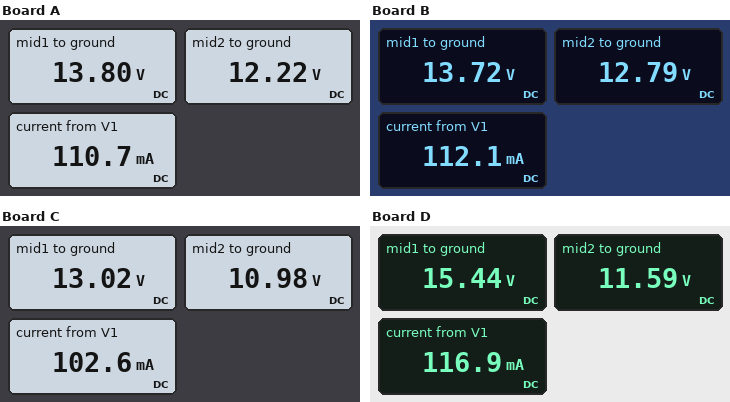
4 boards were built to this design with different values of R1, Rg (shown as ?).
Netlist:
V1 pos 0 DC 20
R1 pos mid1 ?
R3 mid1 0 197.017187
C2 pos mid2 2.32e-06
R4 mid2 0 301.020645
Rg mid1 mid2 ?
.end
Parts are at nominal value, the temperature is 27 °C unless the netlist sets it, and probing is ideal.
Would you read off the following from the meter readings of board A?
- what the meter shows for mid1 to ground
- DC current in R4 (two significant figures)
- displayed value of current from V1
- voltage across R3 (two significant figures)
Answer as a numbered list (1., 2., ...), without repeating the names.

1. 13.80 V
2. 41 mA
3. 110.7 mA
4. 14 V
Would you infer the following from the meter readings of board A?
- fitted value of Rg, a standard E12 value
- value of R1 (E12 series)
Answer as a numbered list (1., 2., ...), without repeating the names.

1. 39 Ω
2. 56 Ω
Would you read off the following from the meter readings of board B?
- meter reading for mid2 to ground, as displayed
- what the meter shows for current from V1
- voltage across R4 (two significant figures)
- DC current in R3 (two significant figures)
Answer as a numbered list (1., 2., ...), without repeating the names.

1. 12.79 V
2. 112.1 mA
3. 13 V
4. 70 mA
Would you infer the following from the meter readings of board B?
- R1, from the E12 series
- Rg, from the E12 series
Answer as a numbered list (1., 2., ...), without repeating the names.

1. 56 Ω
2. 22 Ω
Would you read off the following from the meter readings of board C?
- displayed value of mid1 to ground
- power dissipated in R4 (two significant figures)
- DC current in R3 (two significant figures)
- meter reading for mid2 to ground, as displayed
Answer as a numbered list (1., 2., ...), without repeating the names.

1. 13.02 V
2. 400 mW
3. 66 mA
4. 10.98 V
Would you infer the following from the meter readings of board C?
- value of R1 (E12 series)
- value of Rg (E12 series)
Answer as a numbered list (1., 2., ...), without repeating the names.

1. 68 Ω
2. 56 Ω
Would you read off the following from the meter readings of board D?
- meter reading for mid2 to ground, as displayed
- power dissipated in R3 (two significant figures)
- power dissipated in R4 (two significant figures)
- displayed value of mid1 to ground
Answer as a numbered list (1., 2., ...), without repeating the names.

1. 11.59 V
2. 1.2 W
3. 450 mW
4. 15.44 V
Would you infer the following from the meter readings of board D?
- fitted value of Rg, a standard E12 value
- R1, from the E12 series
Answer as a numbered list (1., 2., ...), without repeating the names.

1. 100 Ω
2. 39 Ω
